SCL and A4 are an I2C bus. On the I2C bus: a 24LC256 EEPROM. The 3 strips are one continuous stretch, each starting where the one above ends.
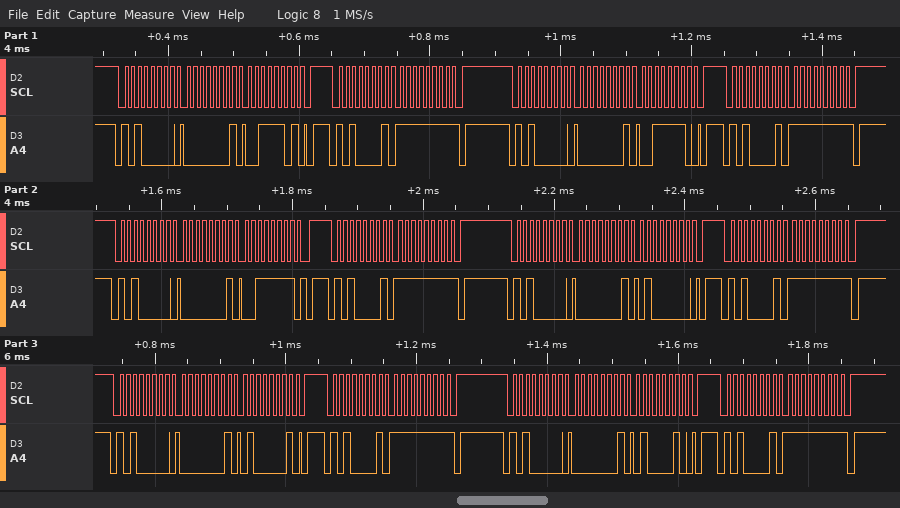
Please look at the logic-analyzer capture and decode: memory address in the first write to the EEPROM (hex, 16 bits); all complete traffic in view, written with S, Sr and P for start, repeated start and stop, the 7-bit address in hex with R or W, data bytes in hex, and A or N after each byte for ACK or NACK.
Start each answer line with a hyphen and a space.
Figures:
- 0x013D
- S 50W A 01 A 3D A P S 50R A FF N P S 50W A 01 A 3E A P S 50R A FF N P S 50W A 01 A 3F A P S 50R A FF N P S 50W A 01 A 40 A P S 50R A FF N P S 50W A 01 A 41 A P S 50R A FF N P S 50W A 01 A 42 A P S 50R A FF N P
